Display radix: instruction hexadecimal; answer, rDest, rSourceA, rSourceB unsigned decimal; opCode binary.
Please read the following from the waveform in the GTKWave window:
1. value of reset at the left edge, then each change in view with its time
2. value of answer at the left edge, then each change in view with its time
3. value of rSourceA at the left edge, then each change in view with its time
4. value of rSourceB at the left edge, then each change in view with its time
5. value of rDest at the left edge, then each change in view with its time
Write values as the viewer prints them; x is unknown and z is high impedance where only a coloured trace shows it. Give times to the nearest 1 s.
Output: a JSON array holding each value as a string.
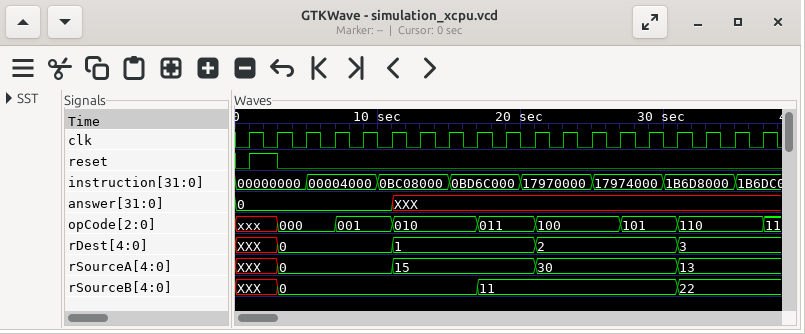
["0, 1 at 1 s, 0 at 3 s", "0, XXX at 11 s", "XXX, 0 at 3 s, 15 at 11 s, 30 at 21 s, 13 at 31 s", "XXX, 0 at 3 s, 11 at 17 s, 22 at 31 s", "XXX, 0 at 3 s, 1 at 11 s, 2 at 21 s, 3 at 31 s"]
